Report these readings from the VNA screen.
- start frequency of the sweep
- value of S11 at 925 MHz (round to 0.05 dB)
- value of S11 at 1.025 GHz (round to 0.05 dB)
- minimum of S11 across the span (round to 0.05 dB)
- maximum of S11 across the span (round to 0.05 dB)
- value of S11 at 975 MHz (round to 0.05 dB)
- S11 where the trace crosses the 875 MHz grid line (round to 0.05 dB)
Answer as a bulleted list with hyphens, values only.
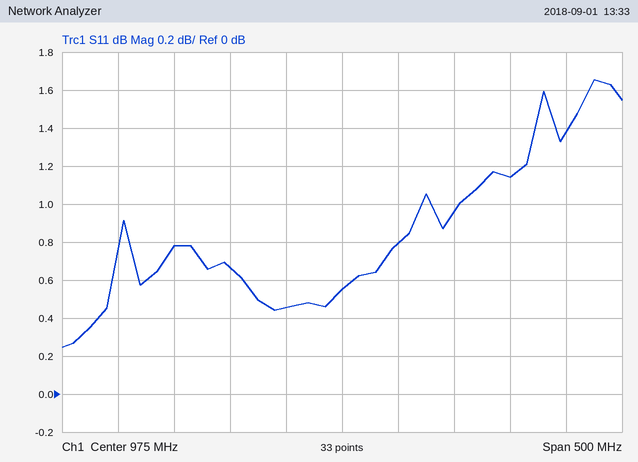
- 725 MHz
- 0.45 dB
- 0.80 dB
- 0.25 dB
- 1.65 dB
- 0.55 dB
- 0.65 dB
